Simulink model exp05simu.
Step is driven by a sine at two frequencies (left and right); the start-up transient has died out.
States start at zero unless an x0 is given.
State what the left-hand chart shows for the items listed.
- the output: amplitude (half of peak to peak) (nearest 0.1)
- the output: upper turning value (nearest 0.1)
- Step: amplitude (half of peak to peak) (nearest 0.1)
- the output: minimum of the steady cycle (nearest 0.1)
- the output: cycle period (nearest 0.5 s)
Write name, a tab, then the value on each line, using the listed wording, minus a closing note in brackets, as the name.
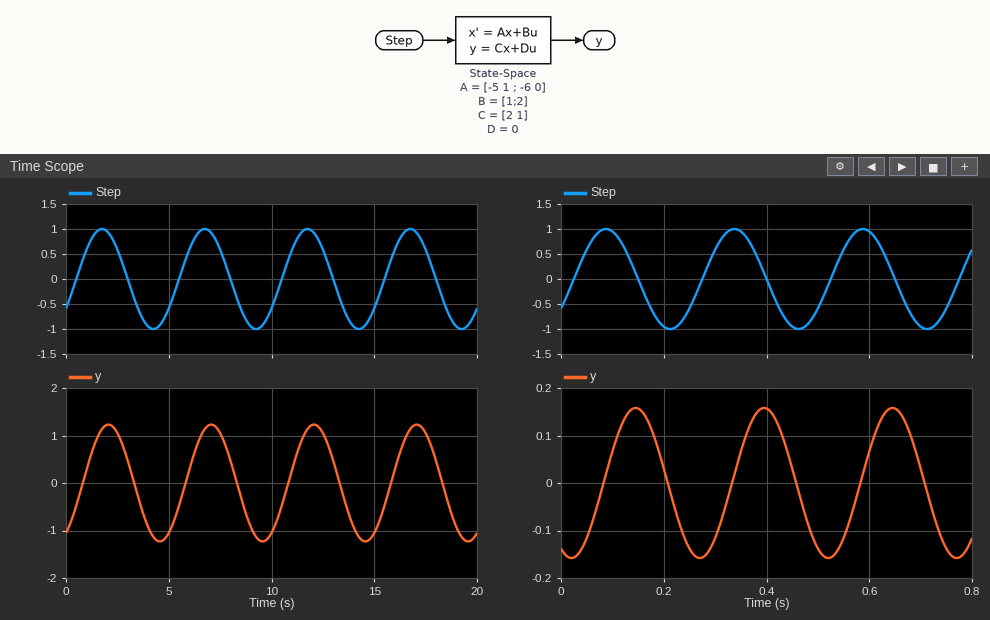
the output: amplitude (half of peak to peak)	1.2
the output: upper turning value	1.2
Step: amplitude (half of peak to peak)	1.0
the output: minimum of the steady cycle	-1.2
the output: cycle period	5.0 s
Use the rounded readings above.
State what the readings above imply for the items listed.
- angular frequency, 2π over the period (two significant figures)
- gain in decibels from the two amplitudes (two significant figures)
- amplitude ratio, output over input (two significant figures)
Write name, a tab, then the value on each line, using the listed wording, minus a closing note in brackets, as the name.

angular frequency, 2π over the period	1.3 rad/s
gain in decibels from the two amplitudes	1.6 dB
amplitude ratio, output over input	1.2
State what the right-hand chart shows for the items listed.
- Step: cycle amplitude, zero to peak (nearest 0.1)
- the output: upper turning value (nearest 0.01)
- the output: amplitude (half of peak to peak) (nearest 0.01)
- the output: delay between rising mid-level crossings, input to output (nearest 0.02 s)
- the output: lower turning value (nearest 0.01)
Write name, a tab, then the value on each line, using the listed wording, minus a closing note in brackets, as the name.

Step: cycle amplitude, zero to peak	1.0
the output: upper turning value	0.16
the output: amplitude (half of peak to peak)	0.16
the output: delay between rising mid-level crossings, input to output	0.06 s
the output: lower turning value	-0.16
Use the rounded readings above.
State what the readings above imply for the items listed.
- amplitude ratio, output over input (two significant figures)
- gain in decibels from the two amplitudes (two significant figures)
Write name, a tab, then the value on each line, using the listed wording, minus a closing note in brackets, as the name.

amplitude ratio, output over input	0.16
gain in decibels from the two amplitudes	-16 dB
